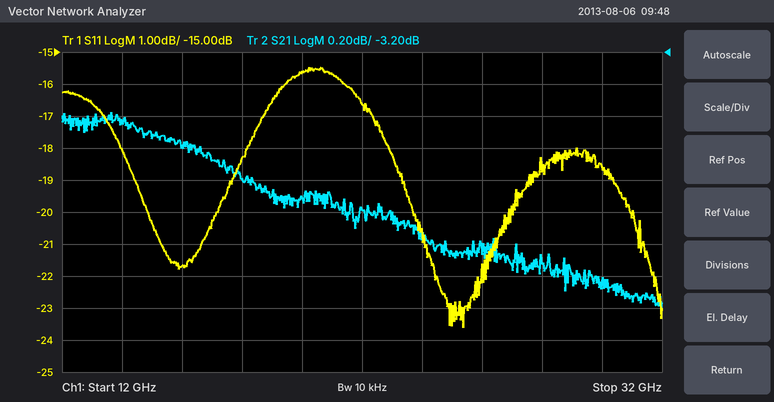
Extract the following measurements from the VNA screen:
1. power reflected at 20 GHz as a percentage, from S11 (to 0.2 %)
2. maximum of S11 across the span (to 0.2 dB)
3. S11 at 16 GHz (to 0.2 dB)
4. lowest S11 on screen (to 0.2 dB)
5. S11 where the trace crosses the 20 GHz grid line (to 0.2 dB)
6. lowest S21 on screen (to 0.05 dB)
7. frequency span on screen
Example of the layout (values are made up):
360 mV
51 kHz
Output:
2.8 %
-15.4 dB
-21.6 dB
-23.6 dB
-15.6 dB
-4.80 dB
20 GHz
